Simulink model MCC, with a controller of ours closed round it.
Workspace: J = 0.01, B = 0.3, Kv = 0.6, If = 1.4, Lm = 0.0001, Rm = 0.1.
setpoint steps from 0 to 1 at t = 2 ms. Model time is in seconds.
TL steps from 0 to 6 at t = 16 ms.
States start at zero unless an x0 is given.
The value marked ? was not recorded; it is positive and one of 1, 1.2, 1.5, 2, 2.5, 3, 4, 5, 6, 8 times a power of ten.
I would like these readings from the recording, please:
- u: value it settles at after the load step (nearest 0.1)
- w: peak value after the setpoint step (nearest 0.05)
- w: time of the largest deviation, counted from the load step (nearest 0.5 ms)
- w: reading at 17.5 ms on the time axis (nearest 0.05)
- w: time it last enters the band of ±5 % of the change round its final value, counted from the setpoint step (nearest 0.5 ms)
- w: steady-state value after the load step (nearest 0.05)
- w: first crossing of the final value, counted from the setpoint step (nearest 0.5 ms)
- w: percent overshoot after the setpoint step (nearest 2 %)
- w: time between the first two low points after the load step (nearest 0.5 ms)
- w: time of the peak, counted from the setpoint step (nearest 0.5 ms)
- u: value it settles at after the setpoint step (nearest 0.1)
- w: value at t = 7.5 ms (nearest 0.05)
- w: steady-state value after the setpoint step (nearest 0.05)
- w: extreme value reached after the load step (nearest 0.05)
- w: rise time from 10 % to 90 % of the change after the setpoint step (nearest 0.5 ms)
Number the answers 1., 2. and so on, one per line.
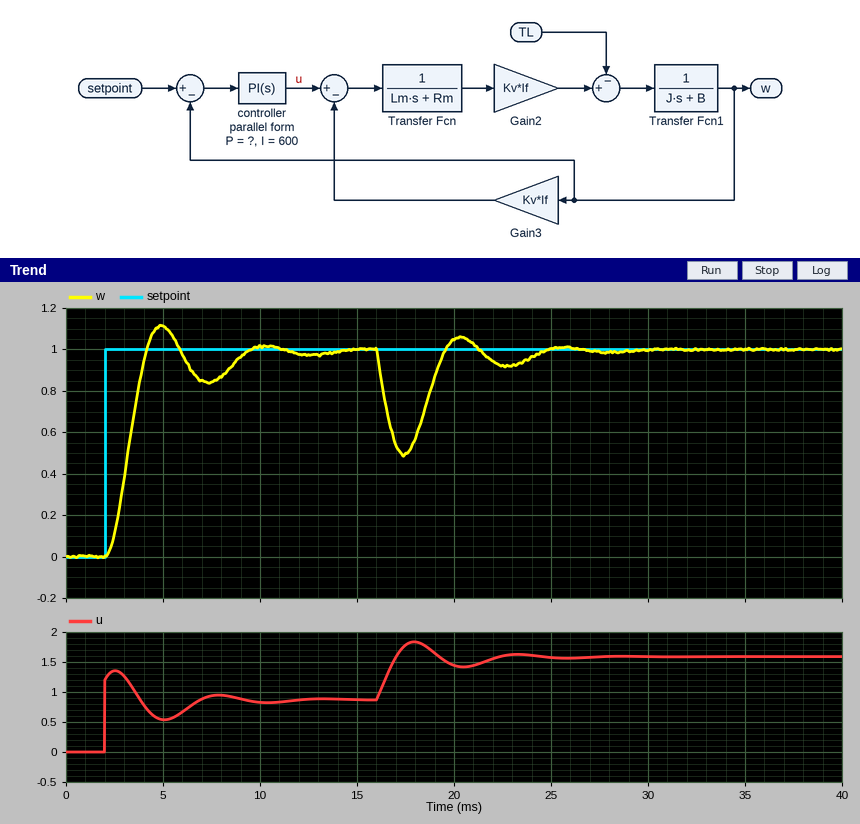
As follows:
1. 1.6
2. 1.10
3. 1.5 ms
4. 0.50
5. 7.0 ms
6. 1.00
7. 2.0 ms
8. 12 %
9. 5.5 ms
10. 3.0 ms
11. 0.9
12. 0.85
13. 1.00
14. 0.50
15. 1.5 ms
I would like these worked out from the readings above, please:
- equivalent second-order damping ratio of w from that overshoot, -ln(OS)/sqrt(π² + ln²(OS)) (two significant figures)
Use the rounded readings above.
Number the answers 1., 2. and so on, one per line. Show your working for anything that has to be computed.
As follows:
1. ln(0.12) = -2.120; 2.120 / sqrt(9.870 + 4.496) = 0.56
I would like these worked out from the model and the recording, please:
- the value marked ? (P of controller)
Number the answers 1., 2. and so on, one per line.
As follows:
1. 1.2
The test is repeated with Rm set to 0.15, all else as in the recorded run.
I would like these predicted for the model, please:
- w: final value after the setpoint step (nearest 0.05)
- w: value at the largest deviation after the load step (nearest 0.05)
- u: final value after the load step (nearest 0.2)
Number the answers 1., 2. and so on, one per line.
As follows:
1. 1.00
2. 0.45
3. 2.0
